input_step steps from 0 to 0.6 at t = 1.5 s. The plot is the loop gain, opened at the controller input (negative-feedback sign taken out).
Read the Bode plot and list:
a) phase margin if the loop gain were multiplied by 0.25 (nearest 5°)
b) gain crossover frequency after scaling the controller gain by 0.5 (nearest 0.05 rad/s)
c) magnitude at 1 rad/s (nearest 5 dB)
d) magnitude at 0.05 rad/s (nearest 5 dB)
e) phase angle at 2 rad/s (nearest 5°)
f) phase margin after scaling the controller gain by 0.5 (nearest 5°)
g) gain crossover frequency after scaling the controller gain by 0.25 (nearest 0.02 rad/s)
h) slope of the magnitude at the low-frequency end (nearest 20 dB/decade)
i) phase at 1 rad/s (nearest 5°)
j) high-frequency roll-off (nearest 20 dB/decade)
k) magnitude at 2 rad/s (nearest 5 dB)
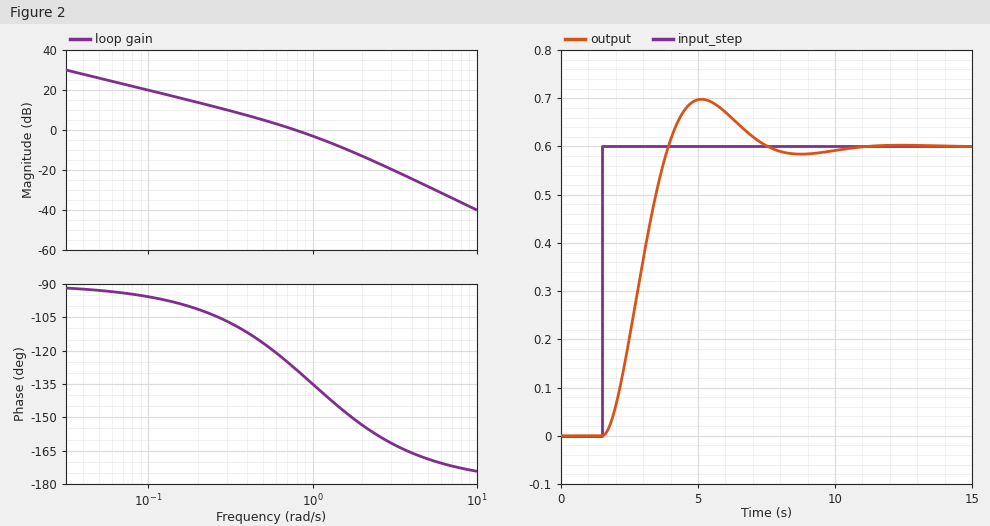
75°
0.45 rad/s
-5 dB
25 dB
-155°
65°
0.24 rad/s
-20 dB/decade
-135°
-40 dB/decade
-15 dB
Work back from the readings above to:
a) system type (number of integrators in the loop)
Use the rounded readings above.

1
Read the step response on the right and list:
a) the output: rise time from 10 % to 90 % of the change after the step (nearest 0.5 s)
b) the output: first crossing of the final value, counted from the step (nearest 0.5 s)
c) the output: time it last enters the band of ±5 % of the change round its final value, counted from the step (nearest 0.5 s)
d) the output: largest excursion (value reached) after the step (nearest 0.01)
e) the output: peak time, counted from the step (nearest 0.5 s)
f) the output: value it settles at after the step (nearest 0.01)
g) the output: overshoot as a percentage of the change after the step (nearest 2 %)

1.5 s
2.5 s
5.5 s
0.70
3.5 s
0.60
16 %
